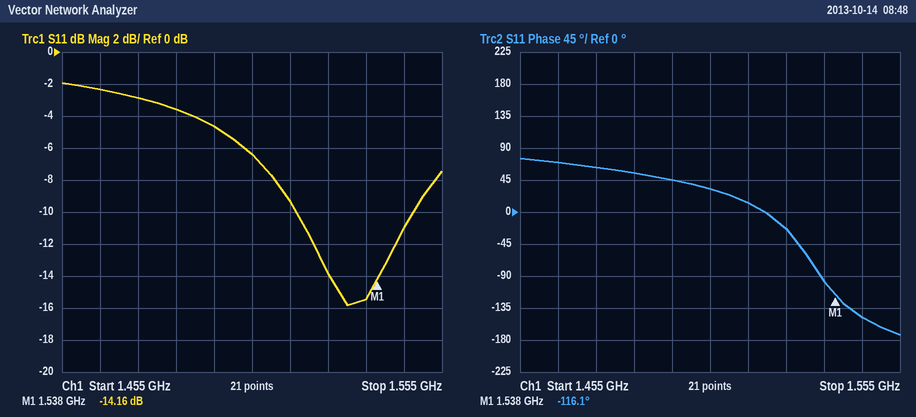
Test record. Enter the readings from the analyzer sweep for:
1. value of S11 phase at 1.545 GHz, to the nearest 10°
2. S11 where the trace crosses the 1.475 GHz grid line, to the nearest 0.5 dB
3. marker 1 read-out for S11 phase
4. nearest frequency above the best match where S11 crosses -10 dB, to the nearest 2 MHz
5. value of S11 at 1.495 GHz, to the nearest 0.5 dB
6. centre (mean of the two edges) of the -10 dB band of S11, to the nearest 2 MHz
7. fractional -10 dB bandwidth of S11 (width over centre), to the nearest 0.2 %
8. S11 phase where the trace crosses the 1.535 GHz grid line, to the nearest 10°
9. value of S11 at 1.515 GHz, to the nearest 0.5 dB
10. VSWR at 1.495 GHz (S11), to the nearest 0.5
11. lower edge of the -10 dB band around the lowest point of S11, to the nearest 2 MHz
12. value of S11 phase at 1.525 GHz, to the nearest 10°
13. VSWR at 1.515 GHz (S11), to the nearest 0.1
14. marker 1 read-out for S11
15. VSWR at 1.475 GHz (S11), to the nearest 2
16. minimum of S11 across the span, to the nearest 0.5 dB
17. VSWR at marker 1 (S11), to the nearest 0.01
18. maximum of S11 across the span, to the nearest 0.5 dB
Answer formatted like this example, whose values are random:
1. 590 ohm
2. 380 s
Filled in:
1. -150°
2. -3.0 dB
3. -116.1°
4. 1.548 GHz
5. -4.5 dB
6. 1.532 GHz
7. 2.0 %
8. -100°
9. -9.5 dB
10. 4.0
11. 1.516 GHz
12. -20°
13. 2.0
14. -14.16 dB
15. 6
16. -16.0 dB
17. 1.49
18. -2.0 dB
